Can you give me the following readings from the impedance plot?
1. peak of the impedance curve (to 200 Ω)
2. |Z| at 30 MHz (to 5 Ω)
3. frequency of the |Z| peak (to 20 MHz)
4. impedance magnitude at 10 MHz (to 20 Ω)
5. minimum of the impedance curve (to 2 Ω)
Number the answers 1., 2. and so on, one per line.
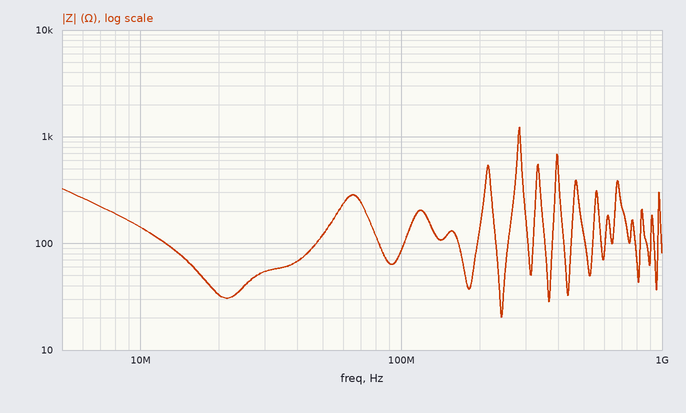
1. 1.2 kΩ
2. 55 Ω
3. 280 MHz
4. 140 Ω
5. 20 Ω
